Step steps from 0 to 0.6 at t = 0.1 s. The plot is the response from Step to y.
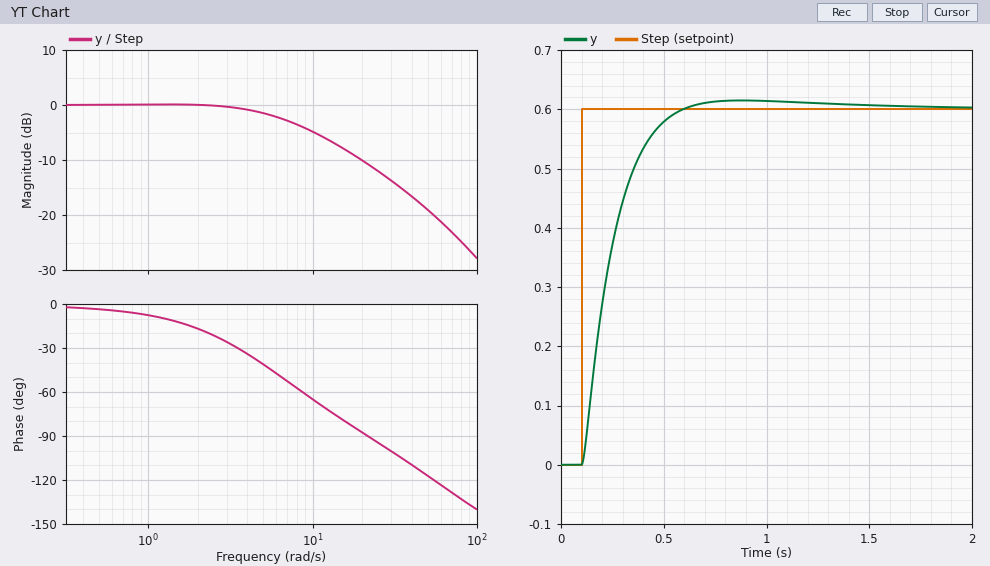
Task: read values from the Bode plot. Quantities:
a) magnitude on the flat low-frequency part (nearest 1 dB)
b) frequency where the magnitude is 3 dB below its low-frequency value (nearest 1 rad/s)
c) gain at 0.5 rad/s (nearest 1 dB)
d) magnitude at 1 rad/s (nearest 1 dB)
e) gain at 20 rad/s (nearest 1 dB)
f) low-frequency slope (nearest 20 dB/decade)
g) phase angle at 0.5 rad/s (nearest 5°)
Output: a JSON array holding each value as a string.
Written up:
["0 dB", "7 rad/s", "0 dB", "0 dB", "-10 dB", "0 dB/decade", "-5°"]
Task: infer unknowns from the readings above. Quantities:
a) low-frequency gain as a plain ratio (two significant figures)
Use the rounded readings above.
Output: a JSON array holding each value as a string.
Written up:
["1.0"]
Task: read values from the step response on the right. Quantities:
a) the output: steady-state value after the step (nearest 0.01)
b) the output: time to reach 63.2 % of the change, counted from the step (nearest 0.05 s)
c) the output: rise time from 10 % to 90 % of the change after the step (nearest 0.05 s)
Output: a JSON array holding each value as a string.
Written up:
["0.60", "0.15 s", "0.30 s"]
